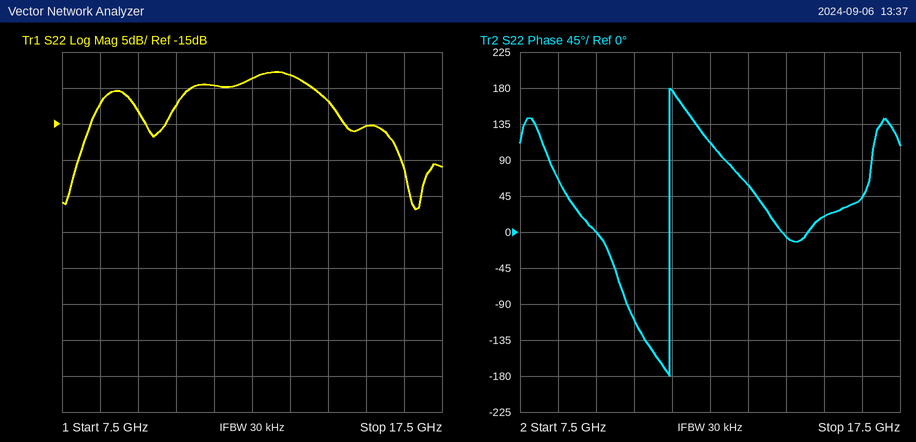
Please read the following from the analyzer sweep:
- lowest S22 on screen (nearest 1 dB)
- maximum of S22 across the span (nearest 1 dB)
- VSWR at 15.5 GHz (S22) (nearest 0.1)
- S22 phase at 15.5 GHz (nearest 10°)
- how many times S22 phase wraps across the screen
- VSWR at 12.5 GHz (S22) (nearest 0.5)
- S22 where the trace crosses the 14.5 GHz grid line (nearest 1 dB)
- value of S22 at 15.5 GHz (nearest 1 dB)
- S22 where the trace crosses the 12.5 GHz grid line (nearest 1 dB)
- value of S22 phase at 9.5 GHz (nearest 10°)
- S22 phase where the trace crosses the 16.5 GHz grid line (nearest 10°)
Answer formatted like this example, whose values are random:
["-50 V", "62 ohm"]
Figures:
["-27 dB", "-8 dB", "1.4", "20°", "1", "2.0", "-12 dB", "-15 dB", "-9 dB", "0°", "40°"]
